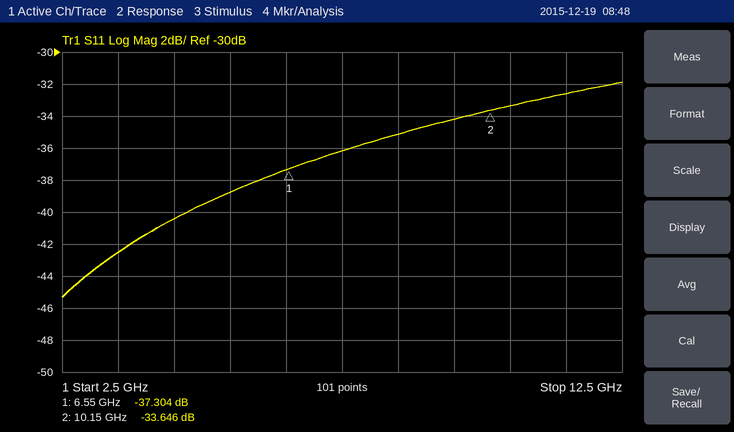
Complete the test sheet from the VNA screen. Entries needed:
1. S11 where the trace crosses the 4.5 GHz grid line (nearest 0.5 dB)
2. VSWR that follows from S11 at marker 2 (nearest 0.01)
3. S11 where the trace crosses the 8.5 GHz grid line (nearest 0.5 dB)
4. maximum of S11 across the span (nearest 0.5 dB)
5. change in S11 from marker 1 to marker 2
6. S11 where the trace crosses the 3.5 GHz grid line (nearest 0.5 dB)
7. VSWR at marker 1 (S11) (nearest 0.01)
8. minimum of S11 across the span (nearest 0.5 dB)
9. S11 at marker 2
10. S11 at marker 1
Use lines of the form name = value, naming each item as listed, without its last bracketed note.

S11 where the trace crosses the 4.5 GHz grid line = -40.5 dB
VSWR that follows from S11 at marker 2 = 1.04
S11 where the trace crosses the 8.5 GHz grid line = -35.0 dB
maximum of S11 across the span = -32.0 dB
change in S11 from marker 1 to marker 2 = 3.658 dB
S11 where the trace crosses the 3.5 GHz grid line = -42.5 dB
VSWR at marker 1 (S11) = 1.03
minimum of S11 across the span = -45.5 dB
S11 at marker 2 = -33.646 dB
S11 at marker 1 = -37.304 dB
